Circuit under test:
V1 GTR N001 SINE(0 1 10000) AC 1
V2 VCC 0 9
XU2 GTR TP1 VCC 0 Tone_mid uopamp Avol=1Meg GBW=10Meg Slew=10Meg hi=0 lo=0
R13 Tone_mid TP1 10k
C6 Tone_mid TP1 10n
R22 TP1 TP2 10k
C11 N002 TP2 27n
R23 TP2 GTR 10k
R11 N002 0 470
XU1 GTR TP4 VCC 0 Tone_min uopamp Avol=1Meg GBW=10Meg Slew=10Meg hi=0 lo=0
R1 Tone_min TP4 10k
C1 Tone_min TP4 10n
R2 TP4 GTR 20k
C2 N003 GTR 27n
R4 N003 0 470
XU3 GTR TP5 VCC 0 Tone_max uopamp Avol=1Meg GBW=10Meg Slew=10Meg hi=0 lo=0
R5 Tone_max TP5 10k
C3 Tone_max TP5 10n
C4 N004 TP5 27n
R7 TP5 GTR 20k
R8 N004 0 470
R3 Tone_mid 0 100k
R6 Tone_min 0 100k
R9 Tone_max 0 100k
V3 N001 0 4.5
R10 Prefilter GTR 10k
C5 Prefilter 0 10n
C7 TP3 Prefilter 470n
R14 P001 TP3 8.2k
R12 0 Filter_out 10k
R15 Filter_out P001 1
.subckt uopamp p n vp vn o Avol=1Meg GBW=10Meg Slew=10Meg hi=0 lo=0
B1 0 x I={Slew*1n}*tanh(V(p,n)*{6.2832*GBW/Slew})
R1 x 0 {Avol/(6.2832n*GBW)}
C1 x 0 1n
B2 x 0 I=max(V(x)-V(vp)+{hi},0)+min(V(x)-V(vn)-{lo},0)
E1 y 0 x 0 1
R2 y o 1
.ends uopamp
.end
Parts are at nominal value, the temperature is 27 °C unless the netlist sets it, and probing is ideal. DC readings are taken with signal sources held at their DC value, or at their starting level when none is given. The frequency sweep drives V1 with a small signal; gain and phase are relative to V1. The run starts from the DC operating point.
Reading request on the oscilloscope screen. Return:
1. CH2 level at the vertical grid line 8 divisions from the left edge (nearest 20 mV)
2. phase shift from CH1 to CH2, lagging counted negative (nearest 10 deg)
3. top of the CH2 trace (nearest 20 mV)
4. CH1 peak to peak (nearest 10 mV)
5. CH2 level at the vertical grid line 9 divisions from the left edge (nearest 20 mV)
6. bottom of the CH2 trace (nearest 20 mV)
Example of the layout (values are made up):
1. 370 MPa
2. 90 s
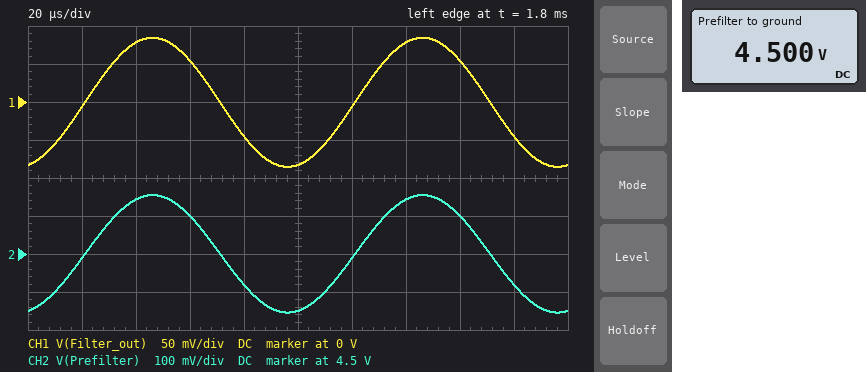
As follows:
1. 4.60 V
2. 0 deg
3. 4.66 V
4. 170 mV
5. 4.42 V
6. 4.34 V
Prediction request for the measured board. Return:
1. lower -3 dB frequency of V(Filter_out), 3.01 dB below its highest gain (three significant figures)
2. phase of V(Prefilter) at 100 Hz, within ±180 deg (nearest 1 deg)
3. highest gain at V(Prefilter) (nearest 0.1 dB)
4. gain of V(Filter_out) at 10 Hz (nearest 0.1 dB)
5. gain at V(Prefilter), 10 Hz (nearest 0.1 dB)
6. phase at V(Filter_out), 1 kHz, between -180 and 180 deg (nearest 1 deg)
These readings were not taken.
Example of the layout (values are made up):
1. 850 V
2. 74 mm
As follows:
1. 11.9 Hz
2. -6 deg
3. 0 dB
4. -12.9 dB
5. -1.2 dB
6. -21 deg
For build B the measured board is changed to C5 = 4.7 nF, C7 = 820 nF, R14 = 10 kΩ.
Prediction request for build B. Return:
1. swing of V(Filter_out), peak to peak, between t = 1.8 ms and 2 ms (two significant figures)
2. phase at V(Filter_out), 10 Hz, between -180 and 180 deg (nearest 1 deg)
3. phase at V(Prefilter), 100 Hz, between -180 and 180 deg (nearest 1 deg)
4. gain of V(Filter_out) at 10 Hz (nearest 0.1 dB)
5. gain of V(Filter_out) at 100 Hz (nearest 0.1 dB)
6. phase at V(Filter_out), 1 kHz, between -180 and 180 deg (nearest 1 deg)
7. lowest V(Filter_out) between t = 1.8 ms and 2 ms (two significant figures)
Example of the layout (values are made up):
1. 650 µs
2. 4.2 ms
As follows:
1. 300 mV
2. 33 deg
3. -3 deg
4. -11.1 dB
5. -9.6 dB
6. -11 deg
7. -150 mV
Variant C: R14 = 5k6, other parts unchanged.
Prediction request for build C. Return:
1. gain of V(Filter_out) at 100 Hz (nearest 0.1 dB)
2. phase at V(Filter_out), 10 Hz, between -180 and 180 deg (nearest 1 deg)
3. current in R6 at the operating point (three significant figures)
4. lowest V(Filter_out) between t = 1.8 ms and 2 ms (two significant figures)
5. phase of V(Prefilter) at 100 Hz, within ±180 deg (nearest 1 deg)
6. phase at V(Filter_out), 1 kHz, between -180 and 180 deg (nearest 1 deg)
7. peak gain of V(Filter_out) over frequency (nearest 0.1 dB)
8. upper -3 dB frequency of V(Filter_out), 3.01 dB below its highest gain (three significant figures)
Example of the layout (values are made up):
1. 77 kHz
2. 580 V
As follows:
1. -8.3 dB
2. 53 deg
3. 45.0 µA
4. -99 mV
5. -7 deg
6. -20 deg
7. -8.2 dB
8. 2.65 kHz
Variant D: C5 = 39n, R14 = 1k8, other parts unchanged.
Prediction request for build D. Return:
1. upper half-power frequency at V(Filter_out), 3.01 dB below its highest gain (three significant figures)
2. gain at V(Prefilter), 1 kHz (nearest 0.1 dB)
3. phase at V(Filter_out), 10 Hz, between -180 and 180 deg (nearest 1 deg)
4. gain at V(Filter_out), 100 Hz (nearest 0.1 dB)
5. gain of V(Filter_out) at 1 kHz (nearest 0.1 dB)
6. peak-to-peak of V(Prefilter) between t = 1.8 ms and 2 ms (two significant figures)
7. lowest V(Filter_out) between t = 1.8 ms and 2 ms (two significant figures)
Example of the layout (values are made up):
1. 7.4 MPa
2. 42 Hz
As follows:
1. 797 Hz
2. -9.8 dB
3. 56 deg
4. -7.1 dB
5. -11.2 dB
6. 81 mV
7. -35 mV
